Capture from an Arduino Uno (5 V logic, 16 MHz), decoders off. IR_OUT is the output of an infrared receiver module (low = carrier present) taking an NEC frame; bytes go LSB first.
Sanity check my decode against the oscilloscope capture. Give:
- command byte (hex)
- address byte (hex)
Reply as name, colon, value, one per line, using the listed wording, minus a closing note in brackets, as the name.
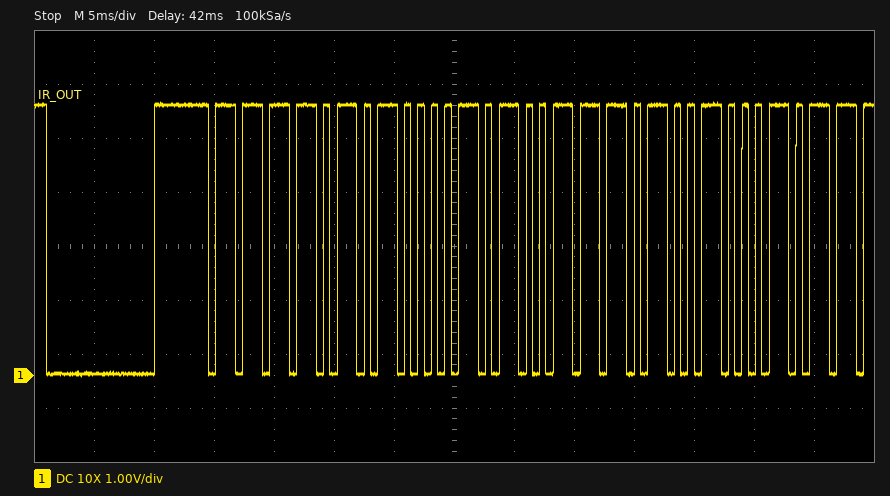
command byte: 0x2E
address byte: 0xAF
